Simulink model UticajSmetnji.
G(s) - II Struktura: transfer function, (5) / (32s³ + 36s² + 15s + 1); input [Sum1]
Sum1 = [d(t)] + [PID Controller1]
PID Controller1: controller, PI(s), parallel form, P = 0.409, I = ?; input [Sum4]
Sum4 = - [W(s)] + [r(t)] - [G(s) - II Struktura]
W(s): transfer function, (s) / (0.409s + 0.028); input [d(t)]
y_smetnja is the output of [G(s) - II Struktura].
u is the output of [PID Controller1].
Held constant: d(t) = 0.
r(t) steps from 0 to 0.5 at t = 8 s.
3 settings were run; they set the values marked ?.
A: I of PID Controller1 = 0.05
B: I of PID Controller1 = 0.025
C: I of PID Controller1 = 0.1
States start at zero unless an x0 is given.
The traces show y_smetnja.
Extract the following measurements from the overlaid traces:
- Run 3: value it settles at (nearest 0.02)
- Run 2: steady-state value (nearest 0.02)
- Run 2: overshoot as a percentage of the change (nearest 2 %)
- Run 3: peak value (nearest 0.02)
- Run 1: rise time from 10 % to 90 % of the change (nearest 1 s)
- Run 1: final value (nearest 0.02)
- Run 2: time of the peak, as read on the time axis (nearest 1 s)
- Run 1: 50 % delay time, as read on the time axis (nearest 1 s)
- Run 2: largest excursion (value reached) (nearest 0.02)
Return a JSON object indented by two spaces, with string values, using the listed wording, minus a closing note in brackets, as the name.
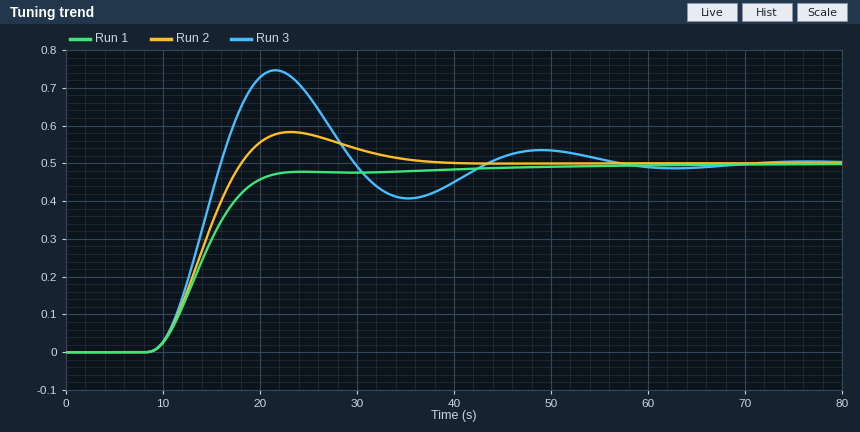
{
  "Run 3: value it settles at": "0.50",
  "Run 2: steady-state value": "0.50",
  "Run 2: overshoot as a percentage of the change": "16 %",
  "Run 3: peak value": "0.74",
  "Run 1: rise time from 10 % to 90 % of the change": "9 s",
  "Run 1: final value": "0.50",
  "Run 2: time of the peak, as read on the time axis": "23 s",
  "Run 1: 50 % delay time, as read on the time axis": "14 s",
  "Run 2: largest excursion (value reached)": "0.58"
}
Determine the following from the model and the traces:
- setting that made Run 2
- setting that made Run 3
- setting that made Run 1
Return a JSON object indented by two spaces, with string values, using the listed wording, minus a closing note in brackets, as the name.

{
  "setting that made Run 2": "A",
  "setting that made Run 3": "C",
  "setting that made Run 1": "B"
}
